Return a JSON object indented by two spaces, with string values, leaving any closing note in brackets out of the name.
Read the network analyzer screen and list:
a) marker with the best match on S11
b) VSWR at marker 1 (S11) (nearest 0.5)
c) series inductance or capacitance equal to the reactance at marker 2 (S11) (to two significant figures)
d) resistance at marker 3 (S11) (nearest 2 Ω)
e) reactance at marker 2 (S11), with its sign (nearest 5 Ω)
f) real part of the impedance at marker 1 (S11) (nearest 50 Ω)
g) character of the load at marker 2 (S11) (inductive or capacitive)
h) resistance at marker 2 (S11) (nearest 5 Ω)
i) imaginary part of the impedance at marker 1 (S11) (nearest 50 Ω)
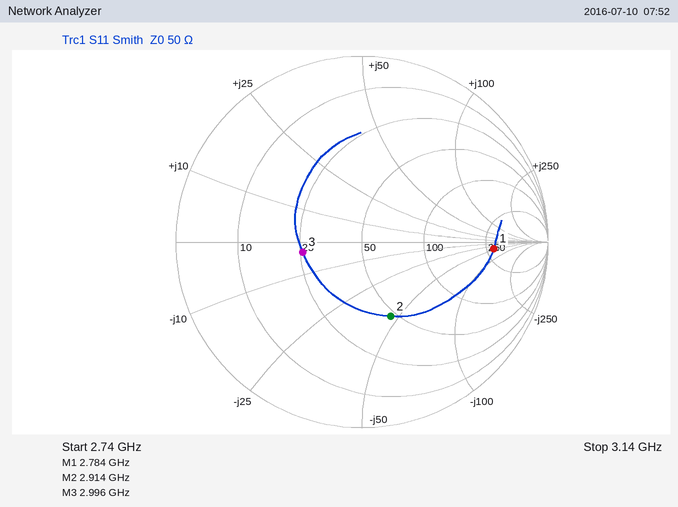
{
  "marker with the best match on S11": "marker 3",
  "VSWR at marker 1 (S11)": "6.0",
  "series inductance or capacitance equal to the reactance at marker 2 (S11)": "1.2 pF",
  "resistance at marker 3 (S11)": "26 Ω",
  "reactance at marker 2 (S11), with its sign": "-45 Ω",
  "real part of the impedance at marker 1 (S11)": "300 Ω",
  "character of the load at marker 2 (S11)": "capacitive",
  "resistance at marker 2 (S11)": "45 Ω",
  "imaginary part of the impedance at marker 1 (S11)": "-50 Ω"
}
